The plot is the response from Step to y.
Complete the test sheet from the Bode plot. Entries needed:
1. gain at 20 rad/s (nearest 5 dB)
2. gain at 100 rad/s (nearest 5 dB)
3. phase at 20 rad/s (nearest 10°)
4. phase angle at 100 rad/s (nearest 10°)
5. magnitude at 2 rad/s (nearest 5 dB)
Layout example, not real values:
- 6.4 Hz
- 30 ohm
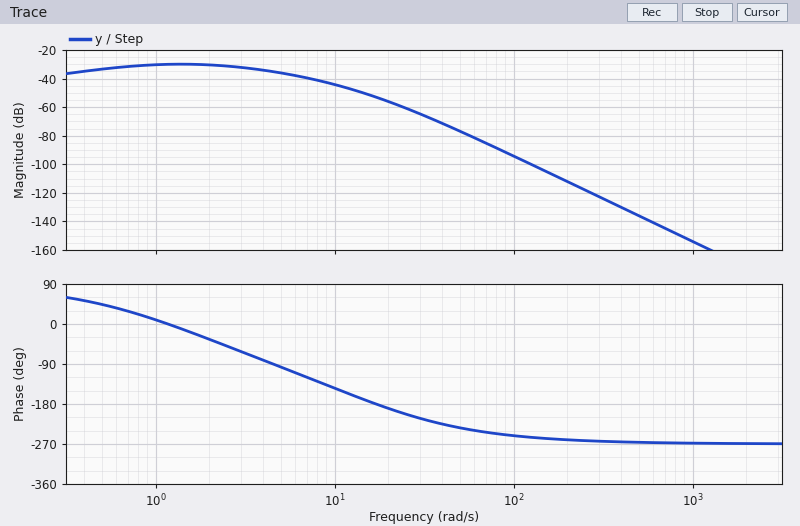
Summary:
- -55 dB
- -95 dB
- -190°
- -250°
- -30 dB
